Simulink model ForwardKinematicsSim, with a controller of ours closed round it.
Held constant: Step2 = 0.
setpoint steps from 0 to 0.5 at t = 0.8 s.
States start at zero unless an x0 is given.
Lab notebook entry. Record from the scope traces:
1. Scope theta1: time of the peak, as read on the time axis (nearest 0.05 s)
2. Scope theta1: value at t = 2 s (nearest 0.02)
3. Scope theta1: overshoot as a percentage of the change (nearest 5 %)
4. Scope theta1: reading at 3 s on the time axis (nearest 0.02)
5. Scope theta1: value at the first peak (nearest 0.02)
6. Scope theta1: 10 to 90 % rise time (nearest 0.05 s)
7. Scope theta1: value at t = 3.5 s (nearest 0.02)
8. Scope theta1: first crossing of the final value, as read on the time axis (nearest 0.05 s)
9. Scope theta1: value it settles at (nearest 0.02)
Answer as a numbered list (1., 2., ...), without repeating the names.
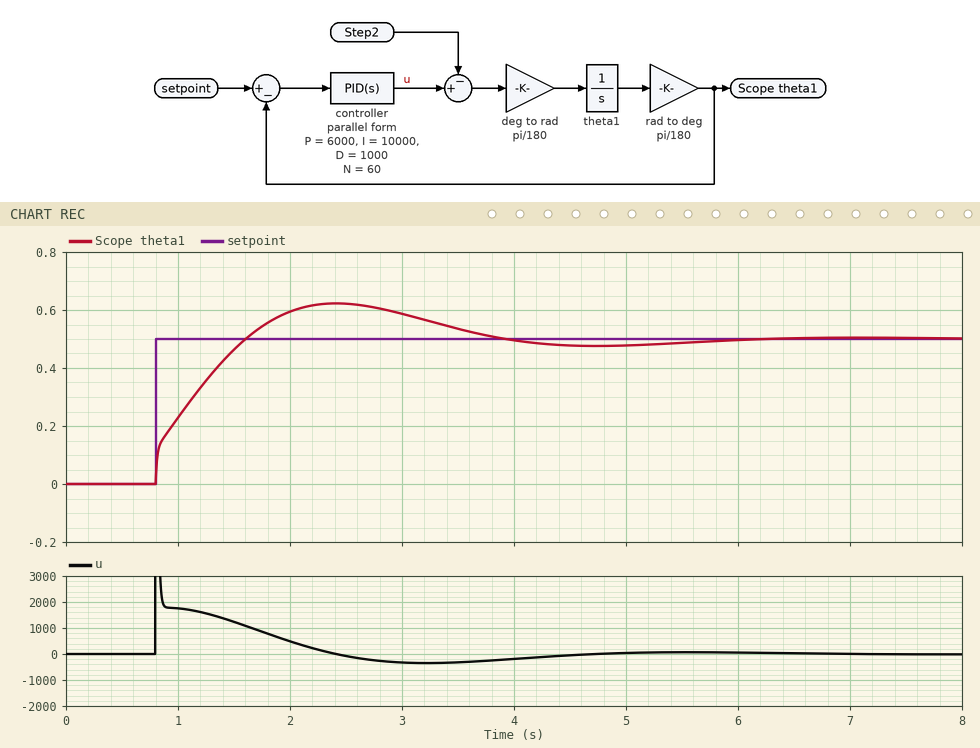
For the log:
1. 2.40 s
2. 0.60
3. 25 %
4. 0.58
5. 0.62
6. 0.65 s
7. 0.54
8. 1.60 s
9. 0.50
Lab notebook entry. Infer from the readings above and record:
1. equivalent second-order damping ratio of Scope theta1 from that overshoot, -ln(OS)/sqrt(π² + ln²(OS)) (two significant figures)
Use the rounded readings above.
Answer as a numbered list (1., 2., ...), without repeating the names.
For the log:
1. 0.40
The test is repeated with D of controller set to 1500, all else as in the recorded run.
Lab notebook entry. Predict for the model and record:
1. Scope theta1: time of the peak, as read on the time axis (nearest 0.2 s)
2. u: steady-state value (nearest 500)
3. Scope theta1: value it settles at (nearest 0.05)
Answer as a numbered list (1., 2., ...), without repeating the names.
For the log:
1. 2.6 s
2. 0
3. 0.50
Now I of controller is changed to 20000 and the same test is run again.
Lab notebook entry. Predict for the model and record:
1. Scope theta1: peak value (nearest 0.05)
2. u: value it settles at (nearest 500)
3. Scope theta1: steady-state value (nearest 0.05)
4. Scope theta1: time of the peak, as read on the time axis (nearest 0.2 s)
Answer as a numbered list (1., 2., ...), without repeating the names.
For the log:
1. 0.65
2. 0
3. 0.50
4. 2.0 s
